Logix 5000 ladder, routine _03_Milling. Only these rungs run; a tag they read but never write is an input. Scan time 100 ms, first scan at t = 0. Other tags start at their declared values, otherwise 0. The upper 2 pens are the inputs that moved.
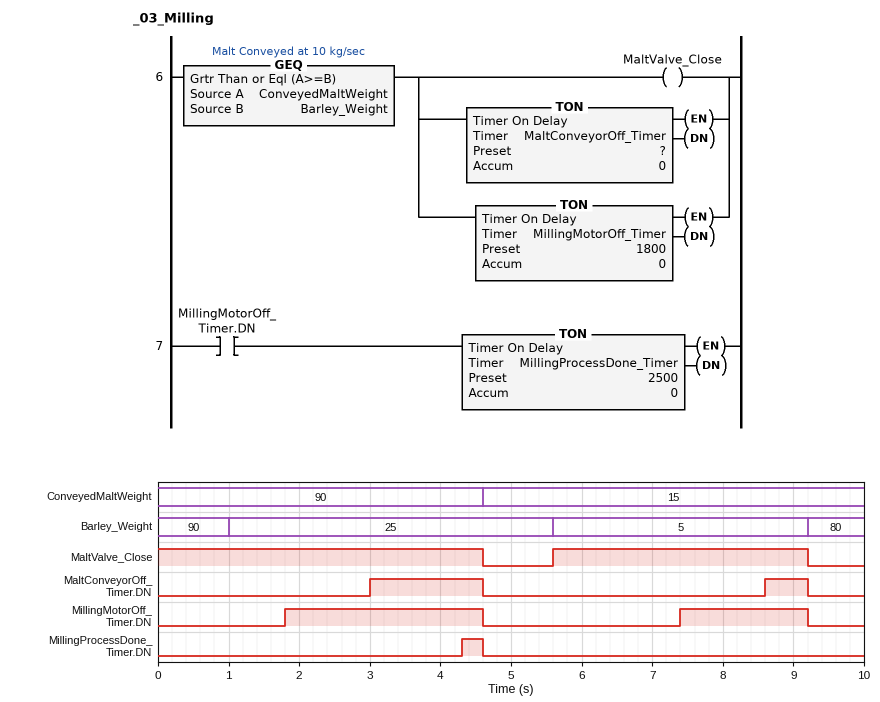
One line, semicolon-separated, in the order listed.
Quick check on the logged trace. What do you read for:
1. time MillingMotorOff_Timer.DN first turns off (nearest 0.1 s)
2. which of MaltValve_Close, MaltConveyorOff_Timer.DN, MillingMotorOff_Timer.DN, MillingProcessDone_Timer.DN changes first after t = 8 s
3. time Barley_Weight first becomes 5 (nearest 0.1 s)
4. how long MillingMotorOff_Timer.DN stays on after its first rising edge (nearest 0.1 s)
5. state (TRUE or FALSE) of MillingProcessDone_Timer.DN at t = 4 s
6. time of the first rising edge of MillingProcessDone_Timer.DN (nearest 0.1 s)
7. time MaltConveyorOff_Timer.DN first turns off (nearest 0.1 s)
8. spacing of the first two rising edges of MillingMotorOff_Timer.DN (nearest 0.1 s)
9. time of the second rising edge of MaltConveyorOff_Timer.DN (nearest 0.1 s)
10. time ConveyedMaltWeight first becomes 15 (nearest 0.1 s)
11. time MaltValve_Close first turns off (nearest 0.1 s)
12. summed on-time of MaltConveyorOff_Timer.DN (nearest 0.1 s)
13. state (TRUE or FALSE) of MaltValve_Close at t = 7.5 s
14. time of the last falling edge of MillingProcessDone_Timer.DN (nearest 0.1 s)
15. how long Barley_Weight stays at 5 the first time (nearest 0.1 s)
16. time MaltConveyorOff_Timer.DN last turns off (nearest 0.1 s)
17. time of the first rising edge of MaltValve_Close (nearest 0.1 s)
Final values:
4.6 s; MaltConveyorOff_Timer.DN; 5.6 s; 2.8 s; FALSE; 4.3 s; 4.6 s; 5.6 s; 8.6 s; 4.6 s; 4.6 s; 2.2 s; TRUE; 4.6 s; 3.6 s; 9.2 s; 5.6 s
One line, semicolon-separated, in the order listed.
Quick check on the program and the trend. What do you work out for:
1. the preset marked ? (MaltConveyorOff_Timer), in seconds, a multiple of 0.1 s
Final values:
3.0 s
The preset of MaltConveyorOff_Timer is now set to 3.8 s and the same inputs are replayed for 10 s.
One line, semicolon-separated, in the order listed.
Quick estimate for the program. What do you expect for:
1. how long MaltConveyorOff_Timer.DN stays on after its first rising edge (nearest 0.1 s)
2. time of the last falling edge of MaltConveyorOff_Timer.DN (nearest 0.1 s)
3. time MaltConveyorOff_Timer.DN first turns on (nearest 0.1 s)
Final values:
0.8 s; 4.6 s; 3.8 s
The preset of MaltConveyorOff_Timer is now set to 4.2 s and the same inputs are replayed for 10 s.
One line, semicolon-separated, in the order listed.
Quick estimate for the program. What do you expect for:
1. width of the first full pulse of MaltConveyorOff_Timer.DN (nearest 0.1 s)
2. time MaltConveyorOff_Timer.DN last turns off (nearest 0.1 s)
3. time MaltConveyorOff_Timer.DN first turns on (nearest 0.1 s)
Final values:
0.4 s; 4.6 s; 4.2 s
